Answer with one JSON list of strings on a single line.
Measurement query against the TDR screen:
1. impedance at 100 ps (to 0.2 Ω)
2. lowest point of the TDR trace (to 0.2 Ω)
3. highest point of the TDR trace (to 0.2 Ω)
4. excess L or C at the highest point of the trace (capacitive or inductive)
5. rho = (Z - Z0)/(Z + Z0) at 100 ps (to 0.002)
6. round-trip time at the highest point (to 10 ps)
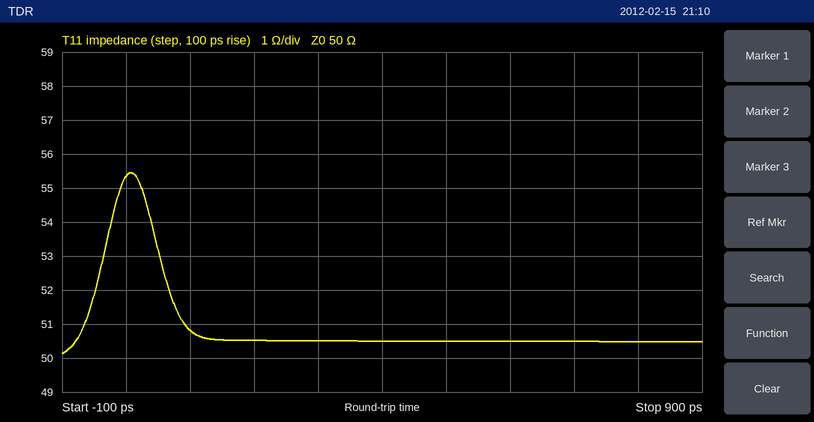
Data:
["50.8 Ω", "50.2 Ω", "55.4 Ω", "inductive", "+0.008", "10 ps"]
